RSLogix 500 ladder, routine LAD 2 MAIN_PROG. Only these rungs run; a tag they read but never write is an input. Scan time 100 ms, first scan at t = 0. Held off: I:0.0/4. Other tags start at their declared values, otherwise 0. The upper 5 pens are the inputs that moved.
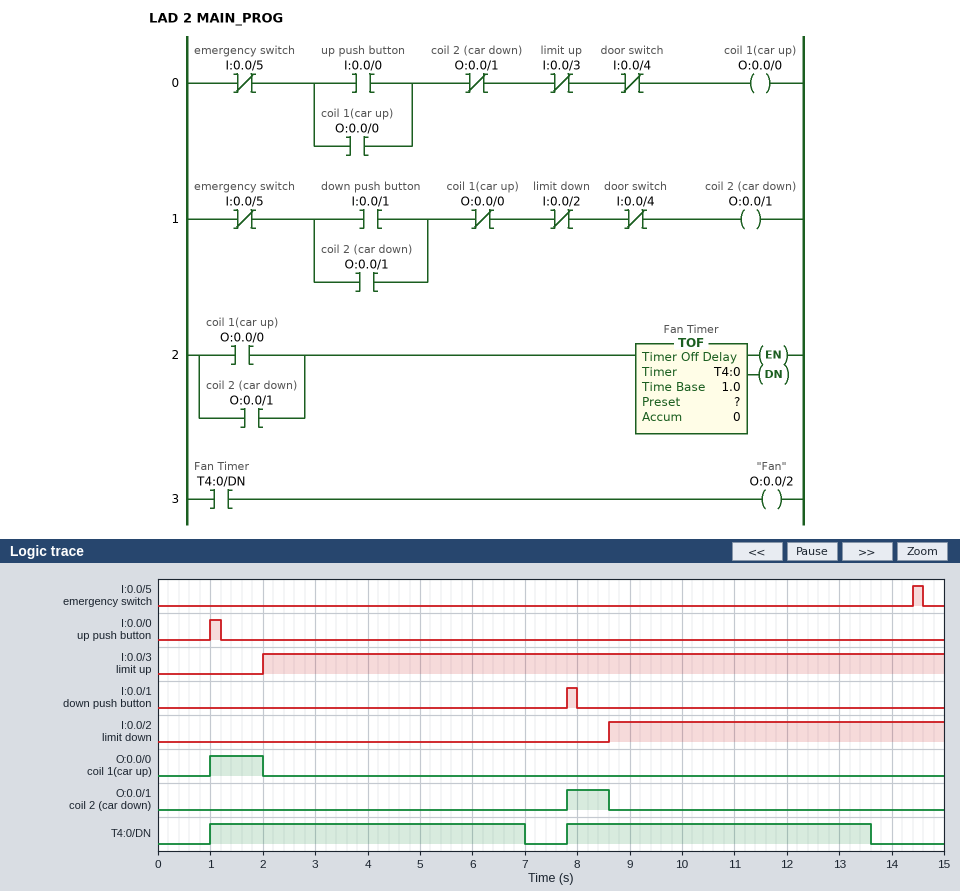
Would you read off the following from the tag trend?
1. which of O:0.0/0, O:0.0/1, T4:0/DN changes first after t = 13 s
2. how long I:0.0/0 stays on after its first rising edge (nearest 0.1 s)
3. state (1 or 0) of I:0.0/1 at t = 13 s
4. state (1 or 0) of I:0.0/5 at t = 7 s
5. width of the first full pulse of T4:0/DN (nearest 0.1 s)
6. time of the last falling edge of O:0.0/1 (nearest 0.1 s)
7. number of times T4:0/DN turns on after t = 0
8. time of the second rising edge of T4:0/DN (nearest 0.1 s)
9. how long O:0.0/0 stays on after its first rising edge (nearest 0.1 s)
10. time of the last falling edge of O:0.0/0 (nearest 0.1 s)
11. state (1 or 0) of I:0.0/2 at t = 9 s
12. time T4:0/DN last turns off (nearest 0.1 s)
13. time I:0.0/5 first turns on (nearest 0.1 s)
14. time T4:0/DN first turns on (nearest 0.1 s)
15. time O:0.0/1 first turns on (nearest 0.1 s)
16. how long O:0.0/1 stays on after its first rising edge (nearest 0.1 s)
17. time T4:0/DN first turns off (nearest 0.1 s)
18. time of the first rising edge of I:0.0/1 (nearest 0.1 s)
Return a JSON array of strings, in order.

["T4:0/DN", "0.2 s", "0", "0", "6.0 s", "8.6 s", "2", "7.8 s", "1.0 s", "2.0 s", "1", "13.6 s", "14.4 s", "1.0 s", "7.8 s", "0.8 s", "7.0 s", "7.8 s"]
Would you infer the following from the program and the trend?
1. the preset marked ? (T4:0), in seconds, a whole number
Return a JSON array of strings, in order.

["5 s"]
